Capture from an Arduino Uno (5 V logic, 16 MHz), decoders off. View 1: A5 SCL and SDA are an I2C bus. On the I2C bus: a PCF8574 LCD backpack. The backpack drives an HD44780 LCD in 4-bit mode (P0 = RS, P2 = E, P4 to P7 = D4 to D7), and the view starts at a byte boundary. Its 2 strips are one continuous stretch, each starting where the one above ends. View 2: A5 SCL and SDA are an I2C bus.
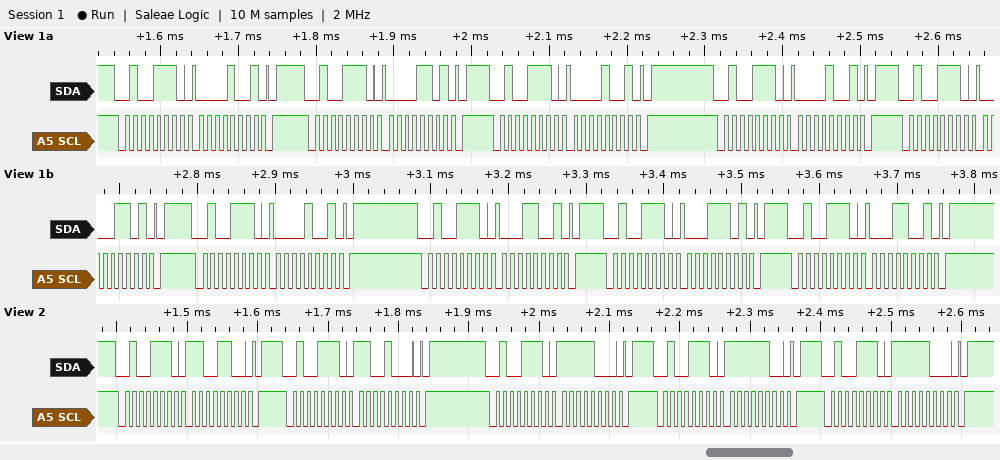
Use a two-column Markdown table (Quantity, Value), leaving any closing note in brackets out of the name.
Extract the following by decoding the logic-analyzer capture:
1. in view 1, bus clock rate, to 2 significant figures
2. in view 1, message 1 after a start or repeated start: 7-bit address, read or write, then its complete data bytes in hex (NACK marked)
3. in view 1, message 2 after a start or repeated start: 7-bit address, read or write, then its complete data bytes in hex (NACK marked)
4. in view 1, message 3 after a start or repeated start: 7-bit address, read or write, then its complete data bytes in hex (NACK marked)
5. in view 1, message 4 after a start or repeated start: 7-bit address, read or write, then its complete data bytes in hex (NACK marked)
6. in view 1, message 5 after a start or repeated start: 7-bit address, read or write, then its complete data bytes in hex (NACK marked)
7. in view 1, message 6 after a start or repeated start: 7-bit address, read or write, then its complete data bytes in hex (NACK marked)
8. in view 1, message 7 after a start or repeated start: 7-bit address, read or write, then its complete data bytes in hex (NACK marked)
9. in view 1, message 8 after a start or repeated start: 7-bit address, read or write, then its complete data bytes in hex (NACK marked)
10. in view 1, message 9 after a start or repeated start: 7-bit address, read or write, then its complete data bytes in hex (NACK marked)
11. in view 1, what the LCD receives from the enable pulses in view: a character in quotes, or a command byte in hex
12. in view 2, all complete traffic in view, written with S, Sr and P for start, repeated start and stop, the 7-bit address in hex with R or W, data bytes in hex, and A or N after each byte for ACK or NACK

| Quantity | Value |
|---|---|
| in view 1, bus clock rate, to 2 significant figures | 100 kHz |
| in view 1, message 1 after a start or repeated start: 7-bit address, read or write, then its complete data bytes in hex | 0x27 write: 09 |
| in view 1, message 2 after a start or repeated start: 7-bit address, read or write, then its complete data bytes in hex | 0x27 write: 0D |
| in view 1, message 3 after a start or repeated start: 7-bit address, read or write, then its complete data bytes in hex | 0x27 write: 09 |
| in view 1, message 4 after a start or repeated start: 7-bit address, read or write, then its complete data bytes in hex | 0x27 write: 09 |
| in view 1, message 5 after a start or repeated start: 7-bit address, read or write, then its complete data bytes in hex | 0x27 write: 0D |
| in view 1, message 6 after a start or repeated start: 7-bit address, read or write, then its complete data bytes in hex | 0x27 write: 09 |
| in view 1, message 7 after a start or repeated start: 7-bit address, read or write, then its complete data bytes in hex | 0x27 write: 19 |
| in view 1, message 8 after a start or repeated start: 7-bit address, read or write, then its complete data bytes in hex | 0x27 write: 1D |
| in view 1, message 9 after a start or repeated start: 7-bit address, read or write, then its complete data bytes in hex | 0x27 write: 19 |
| in view 1, what the LCD receives from the enable pulses in view: a character in quotes, or a command byte in hex | data 0x00 |
| in view 2, all complete traffic in view, written with S, Sr and P for start, repeated start and stop, the 7-bit address in hex with R or W, data bytes in hex, and A or N after each byte for ACK or NACK | S 27W A CC A P S 27W A C8 A P S 27W A F8 A P S 27W A FC A P S 27W A F8 A P |
